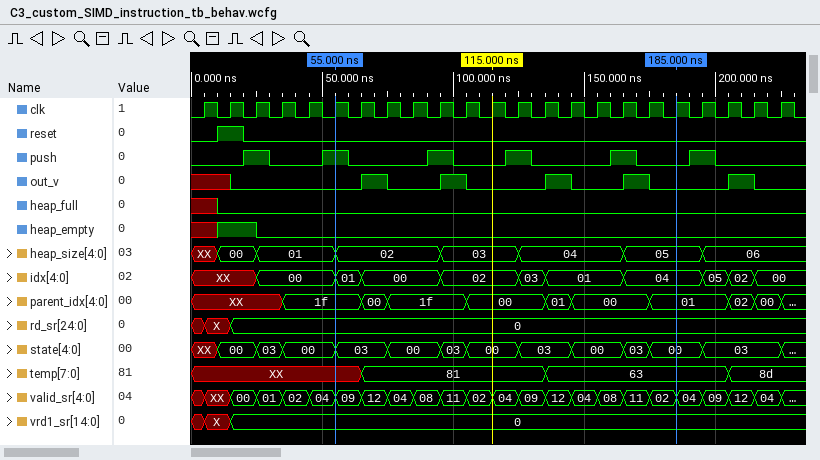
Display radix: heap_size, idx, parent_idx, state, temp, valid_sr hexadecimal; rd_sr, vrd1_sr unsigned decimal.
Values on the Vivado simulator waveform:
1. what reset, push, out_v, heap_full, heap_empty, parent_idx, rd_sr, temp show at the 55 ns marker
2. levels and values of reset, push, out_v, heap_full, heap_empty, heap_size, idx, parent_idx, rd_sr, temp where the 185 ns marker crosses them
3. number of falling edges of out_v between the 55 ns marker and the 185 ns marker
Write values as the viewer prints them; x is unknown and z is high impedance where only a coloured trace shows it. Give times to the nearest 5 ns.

reset=0, push=1, out_v=0, heap_full=0, heap_empty=0, parent_idx=1f, rd_sr=0, temp=XX
reset=0, push=0, out_v=0, heap_full=0, heap_empty=0, heap_size=05, idx=04, parent_idx=01, rd_sr=0, temp=63
4
